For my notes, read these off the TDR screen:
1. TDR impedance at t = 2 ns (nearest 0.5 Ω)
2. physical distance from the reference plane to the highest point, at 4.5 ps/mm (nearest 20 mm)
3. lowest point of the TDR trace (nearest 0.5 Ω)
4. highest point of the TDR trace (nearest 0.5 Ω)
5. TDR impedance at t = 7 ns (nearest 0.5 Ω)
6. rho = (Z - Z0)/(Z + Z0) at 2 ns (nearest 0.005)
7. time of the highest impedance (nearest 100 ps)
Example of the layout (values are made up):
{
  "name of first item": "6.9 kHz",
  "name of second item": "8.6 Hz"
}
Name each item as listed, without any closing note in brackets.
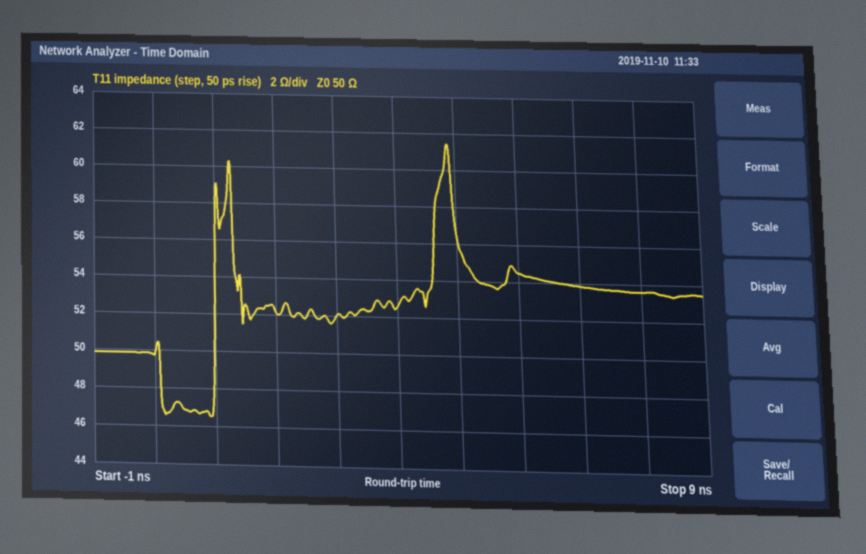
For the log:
{
  "TDR impedance at t = 2 ns": "52.0 Ω",
  "physical distance from the reference plane to the highest point, at 4.5 ps/mm": "540 mm",
  "lowest point of the TDR trace": "46.5 Ω",
  "highest point of the TDR trace": "61.5 Ω",
  "TDR impedance at t = 7 ns": "54.0 Ω",
  "rho = (Z - Z0)/(Z + Z0) at 2 ns": "+0.020",
  "time of the highest impedance": "4.9 ns"
}
